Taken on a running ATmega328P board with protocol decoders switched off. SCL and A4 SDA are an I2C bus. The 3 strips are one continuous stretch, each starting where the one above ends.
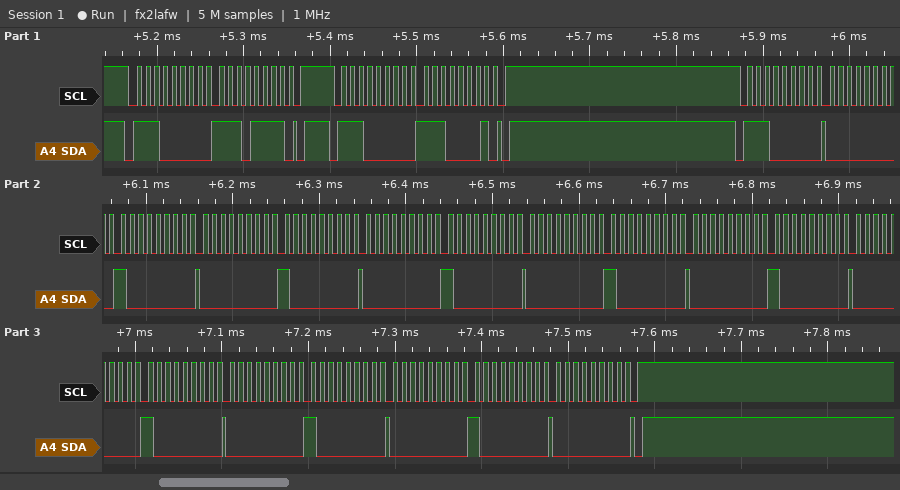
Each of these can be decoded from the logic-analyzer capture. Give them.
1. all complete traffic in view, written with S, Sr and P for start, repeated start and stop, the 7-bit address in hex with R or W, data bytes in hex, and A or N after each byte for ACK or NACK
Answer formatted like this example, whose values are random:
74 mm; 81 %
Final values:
S 70W A EF A P S 70W A E1 A P S 70W A 00 A 80 A 00 A 80 A 00 A 80 A 00 A 80 A 00 A 80 A 00 A 80 A 00 A 80 A 00 A 80 A 00 A P
